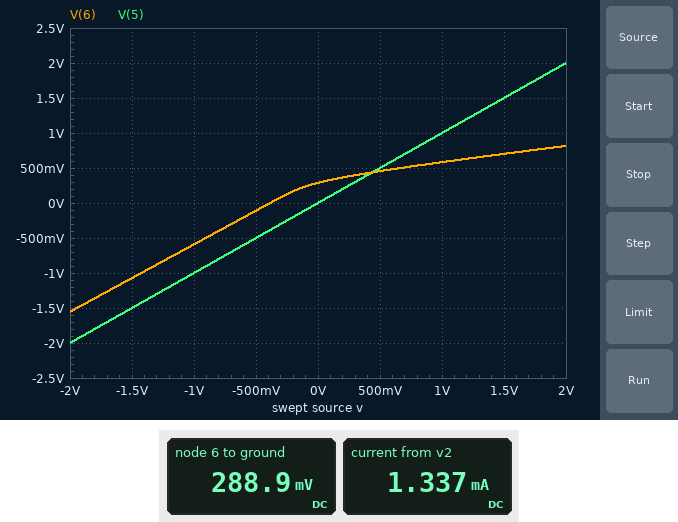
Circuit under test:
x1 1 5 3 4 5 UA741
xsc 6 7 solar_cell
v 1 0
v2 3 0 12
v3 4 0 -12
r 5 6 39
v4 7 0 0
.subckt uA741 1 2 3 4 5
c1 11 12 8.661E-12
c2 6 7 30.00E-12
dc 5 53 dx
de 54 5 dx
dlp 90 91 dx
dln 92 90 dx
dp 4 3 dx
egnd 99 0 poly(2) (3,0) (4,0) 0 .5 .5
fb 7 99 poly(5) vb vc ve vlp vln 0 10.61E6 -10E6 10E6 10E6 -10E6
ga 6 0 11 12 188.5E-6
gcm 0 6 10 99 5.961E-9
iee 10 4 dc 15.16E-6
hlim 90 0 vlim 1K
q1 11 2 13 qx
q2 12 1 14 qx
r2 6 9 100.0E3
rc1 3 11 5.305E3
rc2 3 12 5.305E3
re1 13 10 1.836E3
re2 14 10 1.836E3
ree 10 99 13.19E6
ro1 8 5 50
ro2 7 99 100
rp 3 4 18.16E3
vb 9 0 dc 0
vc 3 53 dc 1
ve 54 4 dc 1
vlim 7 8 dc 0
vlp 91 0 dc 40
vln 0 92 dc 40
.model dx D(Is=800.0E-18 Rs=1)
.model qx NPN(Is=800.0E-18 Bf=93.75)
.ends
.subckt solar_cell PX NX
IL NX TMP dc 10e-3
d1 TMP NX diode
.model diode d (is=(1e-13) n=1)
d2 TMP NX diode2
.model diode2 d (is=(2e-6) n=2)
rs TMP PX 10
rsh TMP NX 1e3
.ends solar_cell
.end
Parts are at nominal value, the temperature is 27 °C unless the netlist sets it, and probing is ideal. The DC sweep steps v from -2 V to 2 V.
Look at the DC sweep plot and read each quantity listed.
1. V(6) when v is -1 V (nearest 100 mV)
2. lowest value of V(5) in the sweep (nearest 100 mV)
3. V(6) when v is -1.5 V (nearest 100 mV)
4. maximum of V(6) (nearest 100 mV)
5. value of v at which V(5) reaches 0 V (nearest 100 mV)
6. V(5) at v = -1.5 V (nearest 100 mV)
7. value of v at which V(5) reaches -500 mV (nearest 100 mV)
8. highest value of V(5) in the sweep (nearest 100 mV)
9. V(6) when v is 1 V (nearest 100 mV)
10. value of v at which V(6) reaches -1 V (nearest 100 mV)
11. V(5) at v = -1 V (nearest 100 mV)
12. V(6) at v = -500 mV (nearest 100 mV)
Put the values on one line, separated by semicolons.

-600 mV; -2.0 V; -1.1 V; 800 mV; 0 V; -1.5 V; -500 mV; 2.0 V; 600 mV; -1.4 V; -1.0 V; -100 mV
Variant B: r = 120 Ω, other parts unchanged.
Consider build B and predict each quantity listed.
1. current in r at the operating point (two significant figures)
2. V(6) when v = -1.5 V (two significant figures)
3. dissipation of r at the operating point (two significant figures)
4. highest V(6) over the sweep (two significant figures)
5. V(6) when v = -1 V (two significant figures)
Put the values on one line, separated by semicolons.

3.2 mA; -280 mV; 1.2 mW; 600 mV; 150 mV
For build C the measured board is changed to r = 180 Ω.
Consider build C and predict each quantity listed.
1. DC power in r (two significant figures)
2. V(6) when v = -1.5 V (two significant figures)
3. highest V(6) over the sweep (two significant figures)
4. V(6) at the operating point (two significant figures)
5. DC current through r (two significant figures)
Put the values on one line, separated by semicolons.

900 µW; 180 mV; 550 mV; 400 mV; 2.2 mA
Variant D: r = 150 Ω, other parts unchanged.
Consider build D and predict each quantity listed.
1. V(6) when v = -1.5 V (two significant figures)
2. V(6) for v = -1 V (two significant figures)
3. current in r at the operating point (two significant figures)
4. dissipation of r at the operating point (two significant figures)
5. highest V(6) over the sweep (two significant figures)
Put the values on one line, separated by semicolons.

-14 mV; 250 mV; 2.6 mA; 1.0 mW; 570 mV
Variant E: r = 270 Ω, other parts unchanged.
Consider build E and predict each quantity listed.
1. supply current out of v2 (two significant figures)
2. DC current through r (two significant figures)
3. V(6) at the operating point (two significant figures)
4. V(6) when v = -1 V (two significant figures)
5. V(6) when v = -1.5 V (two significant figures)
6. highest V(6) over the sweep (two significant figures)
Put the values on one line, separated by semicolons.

1.3 mA; 1.5 mA; 410 mV; 350 mV; 310 mV; 520 mV
